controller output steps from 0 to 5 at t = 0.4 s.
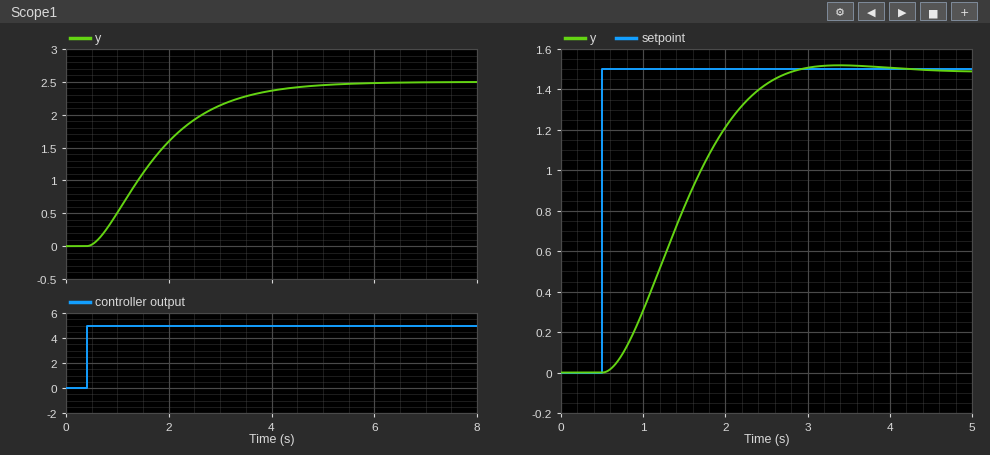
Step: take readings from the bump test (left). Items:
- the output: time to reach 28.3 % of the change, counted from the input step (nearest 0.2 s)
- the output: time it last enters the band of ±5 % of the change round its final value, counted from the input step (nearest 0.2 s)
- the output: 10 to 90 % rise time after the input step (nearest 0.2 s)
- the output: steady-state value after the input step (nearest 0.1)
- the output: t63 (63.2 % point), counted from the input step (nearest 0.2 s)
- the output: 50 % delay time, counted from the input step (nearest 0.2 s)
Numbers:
0.8 s
3.6 s
2.6 s
2.5
1.6 s
1.2 s
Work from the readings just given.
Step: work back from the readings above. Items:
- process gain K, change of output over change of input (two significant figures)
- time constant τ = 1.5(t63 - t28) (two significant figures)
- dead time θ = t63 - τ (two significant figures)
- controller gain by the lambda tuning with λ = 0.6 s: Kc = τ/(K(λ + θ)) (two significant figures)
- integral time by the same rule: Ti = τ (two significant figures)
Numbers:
0.50
1.2 s
0.40 s
2.4
1.2 s
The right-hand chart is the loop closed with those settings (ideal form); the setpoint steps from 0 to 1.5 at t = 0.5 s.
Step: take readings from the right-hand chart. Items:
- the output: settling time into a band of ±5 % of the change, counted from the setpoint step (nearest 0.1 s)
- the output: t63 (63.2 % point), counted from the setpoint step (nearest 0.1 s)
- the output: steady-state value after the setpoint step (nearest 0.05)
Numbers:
2.0 s
1.1 s
1.50
